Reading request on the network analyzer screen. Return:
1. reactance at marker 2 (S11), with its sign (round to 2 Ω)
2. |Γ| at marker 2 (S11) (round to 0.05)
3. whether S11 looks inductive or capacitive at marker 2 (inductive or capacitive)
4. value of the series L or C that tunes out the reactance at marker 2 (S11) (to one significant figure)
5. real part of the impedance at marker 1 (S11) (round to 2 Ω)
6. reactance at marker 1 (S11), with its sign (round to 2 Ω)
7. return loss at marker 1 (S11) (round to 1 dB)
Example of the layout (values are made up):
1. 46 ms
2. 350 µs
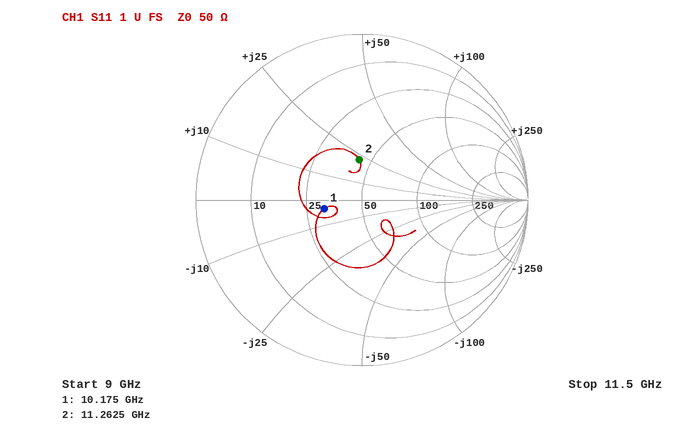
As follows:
1. +22 Ω
2. 0.25
3. inductive
4. 600 fF
5. 32 Ω
6. -4 Ω
7. 13 dB
